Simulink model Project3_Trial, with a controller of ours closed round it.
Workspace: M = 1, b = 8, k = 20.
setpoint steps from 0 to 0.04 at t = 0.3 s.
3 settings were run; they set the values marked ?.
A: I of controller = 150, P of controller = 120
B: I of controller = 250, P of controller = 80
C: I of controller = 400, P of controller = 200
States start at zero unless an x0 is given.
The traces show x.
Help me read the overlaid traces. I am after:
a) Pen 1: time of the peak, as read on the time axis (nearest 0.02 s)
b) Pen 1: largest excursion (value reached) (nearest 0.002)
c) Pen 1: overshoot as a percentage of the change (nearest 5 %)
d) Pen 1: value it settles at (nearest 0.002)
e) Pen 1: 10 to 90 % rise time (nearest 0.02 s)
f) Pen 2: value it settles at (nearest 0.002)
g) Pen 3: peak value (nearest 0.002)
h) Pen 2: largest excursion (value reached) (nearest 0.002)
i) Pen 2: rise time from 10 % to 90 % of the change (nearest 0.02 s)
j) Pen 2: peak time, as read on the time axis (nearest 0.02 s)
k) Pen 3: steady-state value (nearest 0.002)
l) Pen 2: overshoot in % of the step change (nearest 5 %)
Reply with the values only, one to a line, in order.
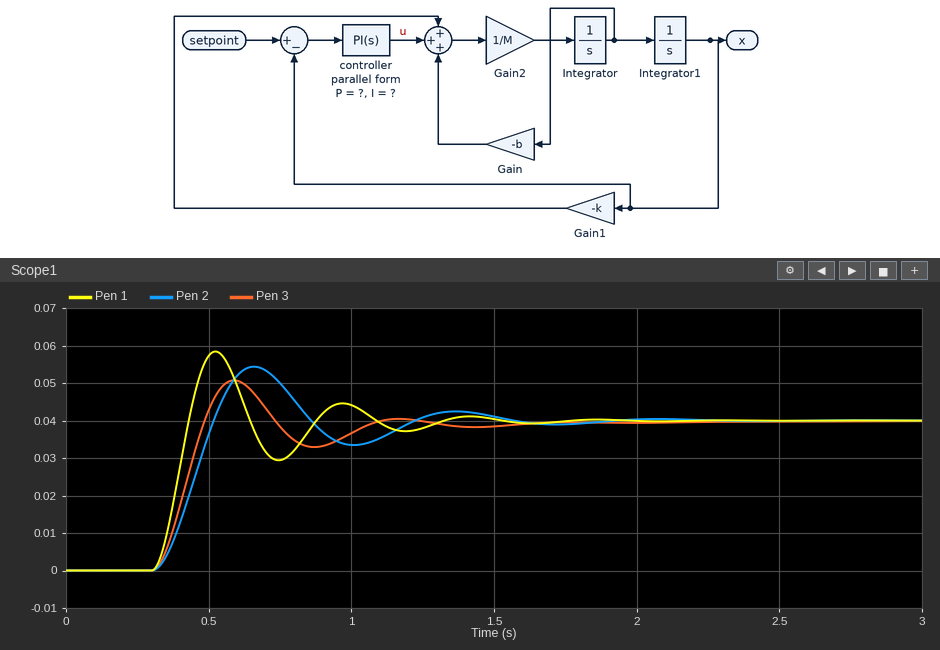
0.52 s
0.058
45 %
0.040
0.08 s
0.040
0.050
0.054
0.14 s
0.66 s
0.040
35 %
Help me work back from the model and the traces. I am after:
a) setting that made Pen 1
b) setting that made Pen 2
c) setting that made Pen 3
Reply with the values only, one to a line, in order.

C
B
A
